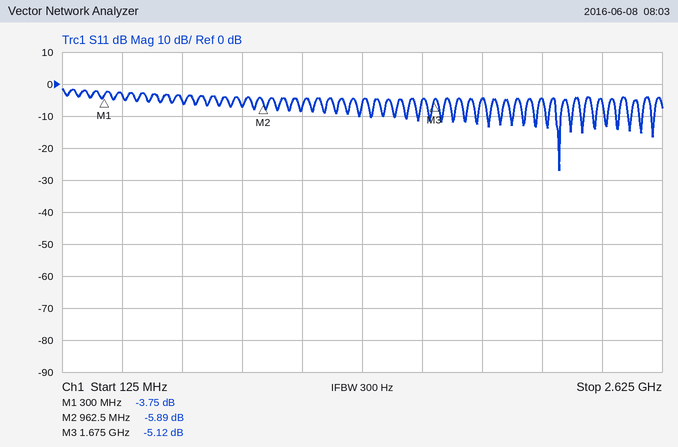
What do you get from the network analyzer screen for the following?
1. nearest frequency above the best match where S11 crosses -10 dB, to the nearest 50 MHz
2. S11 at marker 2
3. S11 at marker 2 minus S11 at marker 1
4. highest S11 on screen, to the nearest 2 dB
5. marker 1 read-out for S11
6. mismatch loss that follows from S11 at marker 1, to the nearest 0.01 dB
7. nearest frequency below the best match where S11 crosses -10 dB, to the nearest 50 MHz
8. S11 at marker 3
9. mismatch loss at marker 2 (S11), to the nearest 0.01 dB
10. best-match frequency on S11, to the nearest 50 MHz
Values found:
2.20 GHz
-5.89 dB
-2.14 dB
-2 dB
-3.75 dB
2.38 dB
2.20 GHz
-5.12 dB
1.29 dB
2.20 GHz
